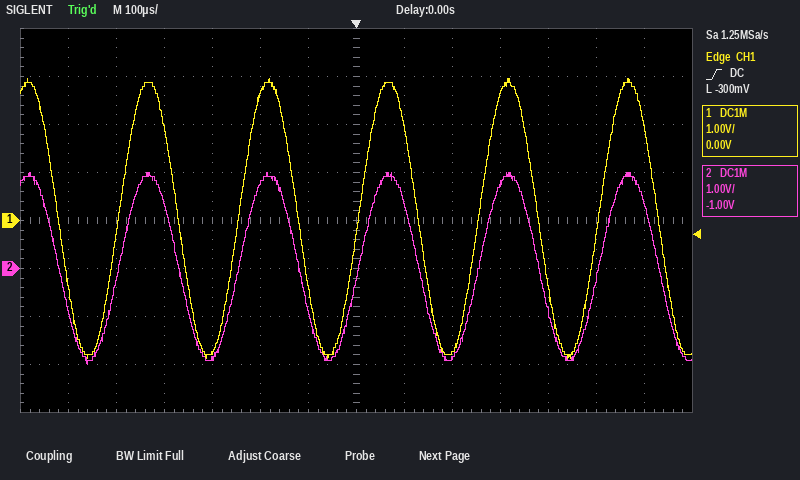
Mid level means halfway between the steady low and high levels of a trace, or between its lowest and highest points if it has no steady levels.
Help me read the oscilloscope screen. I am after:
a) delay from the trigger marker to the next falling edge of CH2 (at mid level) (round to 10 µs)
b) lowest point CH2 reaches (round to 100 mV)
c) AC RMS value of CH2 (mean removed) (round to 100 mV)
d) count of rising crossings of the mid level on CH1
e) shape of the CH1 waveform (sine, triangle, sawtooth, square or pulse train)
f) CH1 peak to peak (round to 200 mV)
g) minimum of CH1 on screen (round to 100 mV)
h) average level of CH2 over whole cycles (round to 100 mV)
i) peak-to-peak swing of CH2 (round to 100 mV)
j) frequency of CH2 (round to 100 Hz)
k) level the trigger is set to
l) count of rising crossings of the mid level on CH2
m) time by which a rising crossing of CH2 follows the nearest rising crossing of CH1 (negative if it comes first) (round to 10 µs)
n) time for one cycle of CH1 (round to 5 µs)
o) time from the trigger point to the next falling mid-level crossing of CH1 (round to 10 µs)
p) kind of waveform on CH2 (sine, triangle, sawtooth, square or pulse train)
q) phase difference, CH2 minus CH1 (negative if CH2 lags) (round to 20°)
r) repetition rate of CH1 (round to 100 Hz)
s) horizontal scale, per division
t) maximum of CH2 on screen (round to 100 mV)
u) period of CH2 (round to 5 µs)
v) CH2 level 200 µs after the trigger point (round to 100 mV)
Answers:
130 µs
-2.0 V
1.4 V
5
sine
5.8 V
-2.9 V
0.0 V
4.0 V
4.0 kHz
-300 mV
5
0 µs
250 µs
130 µs
sine
0°
4.0 kHz
100 µs
2.0 V
250 µs
-1.9 V
